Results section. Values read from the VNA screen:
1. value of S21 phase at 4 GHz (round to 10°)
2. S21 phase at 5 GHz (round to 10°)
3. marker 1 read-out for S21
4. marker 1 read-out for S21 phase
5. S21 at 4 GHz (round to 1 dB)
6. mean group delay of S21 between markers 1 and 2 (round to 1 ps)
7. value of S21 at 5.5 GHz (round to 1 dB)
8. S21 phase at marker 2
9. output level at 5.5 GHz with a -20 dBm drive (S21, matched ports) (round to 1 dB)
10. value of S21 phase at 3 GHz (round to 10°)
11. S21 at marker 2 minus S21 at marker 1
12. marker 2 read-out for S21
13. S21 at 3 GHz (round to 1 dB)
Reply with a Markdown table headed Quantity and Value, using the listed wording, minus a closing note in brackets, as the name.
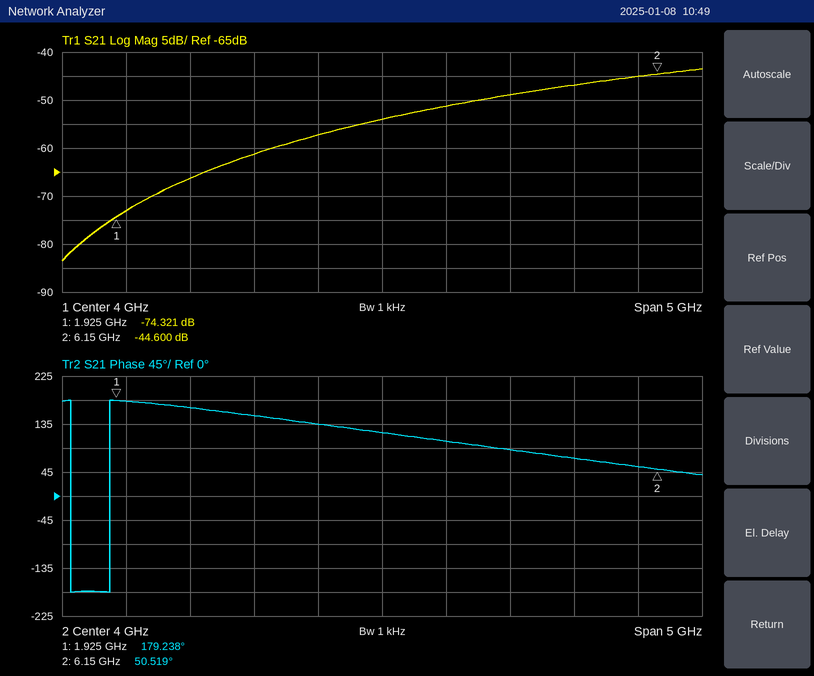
| Quantity | Value |
|---|---|
| value of S21 phase at 4 GHz | 120° |
| S21 phase at 5 GHz | 90° |
| marker 1 read-out for S21 | -74.321 dB |
| marker 1 read-out for S21 phase | 179.238° |
| S21 at 4 GHz | -54 dB |
| mean group delay of S21 between markers 1 and 2 | 85 ps |
| value of S21 at 5.5 GHz | -47 dB |
| S21 phase at marker 2 | 50.519° |
| output level at 5.5 GHz with a -20 dBm drive (S21, matched ports) | -67 dBm |
| value of S21 phase at 3 GHz | 150° |
| S21 at marker 2 minus S21 at marker 1 | 29.721 dB |
| marker 2 read-out for S21 | -44.600 dB |
| S21 at 3 GHz | -61 dB |
